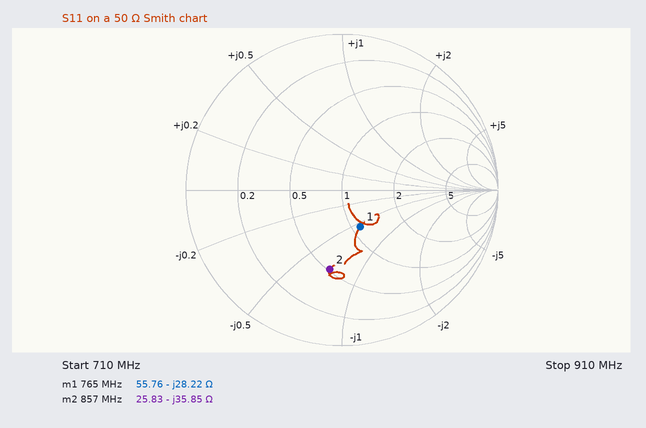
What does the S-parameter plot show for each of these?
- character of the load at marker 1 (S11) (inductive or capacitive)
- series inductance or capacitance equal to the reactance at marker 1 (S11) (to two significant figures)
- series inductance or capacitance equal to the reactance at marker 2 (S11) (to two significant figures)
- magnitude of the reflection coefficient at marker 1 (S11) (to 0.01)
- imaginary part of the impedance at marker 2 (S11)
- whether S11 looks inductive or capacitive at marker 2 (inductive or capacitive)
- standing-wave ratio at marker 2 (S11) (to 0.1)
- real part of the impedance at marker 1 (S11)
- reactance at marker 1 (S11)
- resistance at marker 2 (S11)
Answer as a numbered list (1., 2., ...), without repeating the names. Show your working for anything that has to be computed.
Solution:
1. capacitive
2. C = 1/(2π × 765 MHz × 28.22 Ω) ≈ 7.4 pF
3. C = 1/(2π × 857 MHz × 35.85 Ω) ≈ 5.2 pF
4. 0.26
5. -35.85 Ω
6. capacitive
7. 3.1
8. 55.76 Ω
9. -28.22 Ω
10. 25.83 Ω
